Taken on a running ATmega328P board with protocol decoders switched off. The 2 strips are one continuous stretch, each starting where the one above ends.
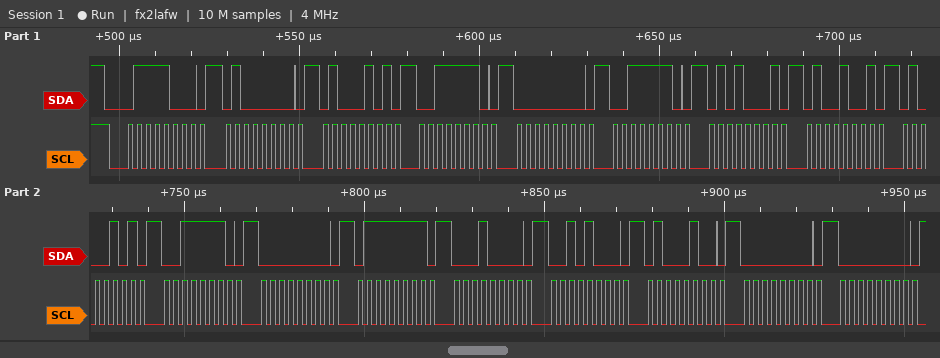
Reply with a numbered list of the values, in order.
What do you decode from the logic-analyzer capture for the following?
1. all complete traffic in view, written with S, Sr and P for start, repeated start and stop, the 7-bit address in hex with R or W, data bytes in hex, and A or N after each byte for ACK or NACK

1. S 3CW A 40 A 45 A 3E A 00 A 3E A 51 A 49 A 45 A 3E A 00 A 7F A 10 A 28 A 44 A 00 A 00 A
